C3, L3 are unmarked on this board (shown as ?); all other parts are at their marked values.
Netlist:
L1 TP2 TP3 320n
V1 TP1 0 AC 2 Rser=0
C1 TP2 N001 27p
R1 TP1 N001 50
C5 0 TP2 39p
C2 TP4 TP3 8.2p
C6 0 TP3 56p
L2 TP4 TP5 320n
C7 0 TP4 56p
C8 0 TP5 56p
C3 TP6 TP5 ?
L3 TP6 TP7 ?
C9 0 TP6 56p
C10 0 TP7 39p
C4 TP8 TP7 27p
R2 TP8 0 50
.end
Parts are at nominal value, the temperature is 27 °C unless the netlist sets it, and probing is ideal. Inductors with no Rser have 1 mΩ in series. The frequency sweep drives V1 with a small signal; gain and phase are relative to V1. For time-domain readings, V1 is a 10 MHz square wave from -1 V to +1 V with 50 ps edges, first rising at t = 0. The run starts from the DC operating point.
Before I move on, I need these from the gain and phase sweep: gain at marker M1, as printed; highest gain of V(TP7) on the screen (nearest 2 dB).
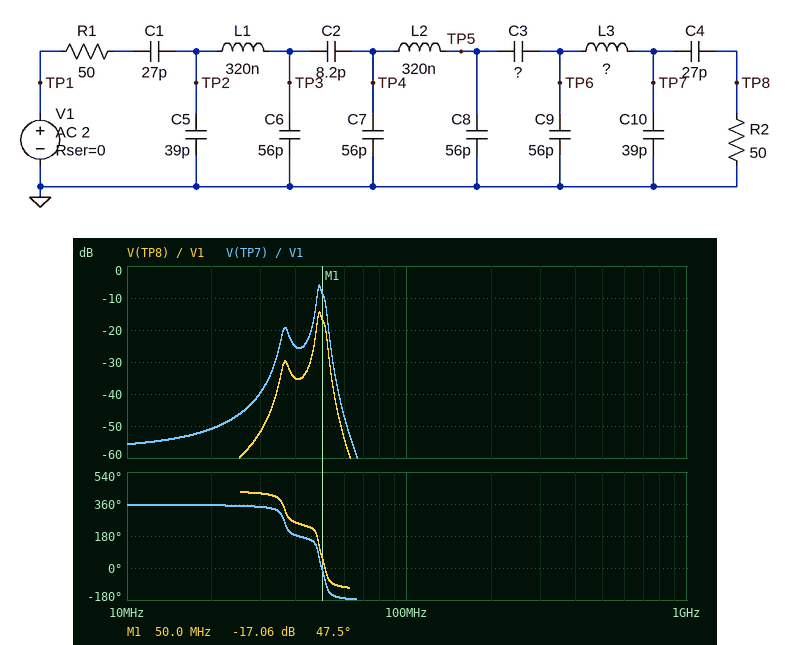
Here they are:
-17.06 dB
-6 dB
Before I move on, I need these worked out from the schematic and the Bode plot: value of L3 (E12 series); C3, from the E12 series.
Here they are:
560 nH
15 pF
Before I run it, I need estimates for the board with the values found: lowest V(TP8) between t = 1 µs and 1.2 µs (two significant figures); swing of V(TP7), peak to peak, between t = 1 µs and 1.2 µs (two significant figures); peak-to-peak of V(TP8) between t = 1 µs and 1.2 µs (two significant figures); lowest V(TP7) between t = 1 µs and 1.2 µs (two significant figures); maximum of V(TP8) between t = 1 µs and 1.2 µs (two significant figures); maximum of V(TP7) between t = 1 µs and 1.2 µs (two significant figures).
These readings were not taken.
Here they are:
-37 mV
190 mV
74 mV
-94 mV
37 mV
97 mV
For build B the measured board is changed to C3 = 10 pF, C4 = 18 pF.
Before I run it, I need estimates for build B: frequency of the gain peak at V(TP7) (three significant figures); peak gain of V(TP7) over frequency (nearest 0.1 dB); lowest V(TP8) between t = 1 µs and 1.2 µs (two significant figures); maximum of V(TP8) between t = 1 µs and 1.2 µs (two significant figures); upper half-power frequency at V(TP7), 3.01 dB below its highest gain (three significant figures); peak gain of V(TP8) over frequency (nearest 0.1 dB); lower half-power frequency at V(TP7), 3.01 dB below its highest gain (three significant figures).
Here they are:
49.0 MHz
-7.5 dB
-26 mV
26 mV
51.3 MHz
-19.0 dB
48.0 MHz
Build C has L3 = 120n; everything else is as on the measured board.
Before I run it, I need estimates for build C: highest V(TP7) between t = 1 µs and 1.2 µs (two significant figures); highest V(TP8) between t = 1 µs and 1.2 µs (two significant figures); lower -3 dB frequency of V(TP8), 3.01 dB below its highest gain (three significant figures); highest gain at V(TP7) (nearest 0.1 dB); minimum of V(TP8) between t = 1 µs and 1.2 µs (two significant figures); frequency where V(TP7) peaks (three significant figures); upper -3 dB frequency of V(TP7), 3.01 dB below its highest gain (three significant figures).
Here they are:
99 mV
38 mV
47.4 MHz
-3.7 dB
-38 mV
48.0 MHz
48.9 MHz
